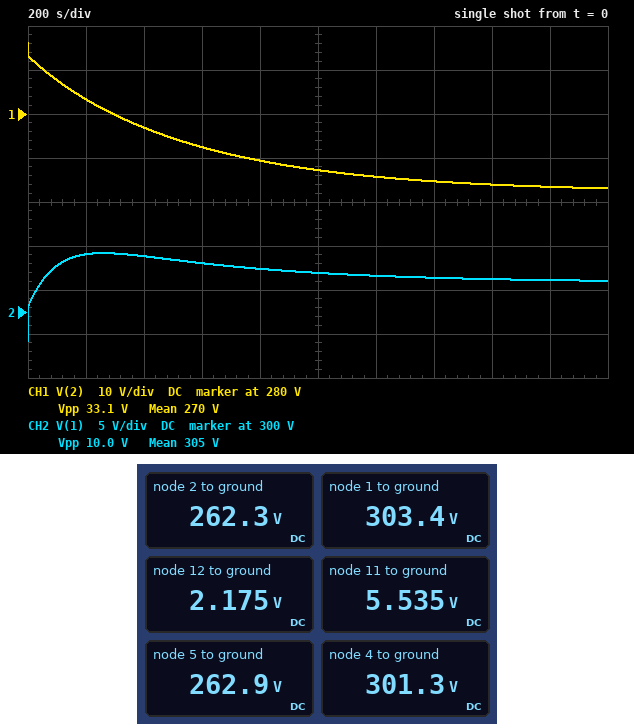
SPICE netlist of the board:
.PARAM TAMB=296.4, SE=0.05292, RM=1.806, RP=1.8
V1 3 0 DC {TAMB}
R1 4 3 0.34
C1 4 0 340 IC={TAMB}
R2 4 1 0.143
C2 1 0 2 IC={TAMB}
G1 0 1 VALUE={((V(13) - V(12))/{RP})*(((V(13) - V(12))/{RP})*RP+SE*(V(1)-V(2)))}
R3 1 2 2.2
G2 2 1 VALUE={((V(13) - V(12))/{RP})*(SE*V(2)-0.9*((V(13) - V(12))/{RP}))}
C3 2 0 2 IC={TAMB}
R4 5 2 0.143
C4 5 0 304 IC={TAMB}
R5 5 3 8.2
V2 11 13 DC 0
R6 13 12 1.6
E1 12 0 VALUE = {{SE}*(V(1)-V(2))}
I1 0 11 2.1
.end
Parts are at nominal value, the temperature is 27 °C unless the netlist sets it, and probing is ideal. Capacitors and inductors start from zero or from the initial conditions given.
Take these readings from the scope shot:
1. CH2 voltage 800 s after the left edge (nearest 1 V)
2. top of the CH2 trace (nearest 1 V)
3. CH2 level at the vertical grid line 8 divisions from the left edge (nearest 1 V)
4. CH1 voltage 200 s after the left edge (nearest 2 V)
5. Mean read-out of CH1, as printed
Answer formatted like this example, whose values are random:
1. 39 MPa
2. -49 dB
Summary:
1. 305 V
2. 307 V
3. 304 V
4. 284 V
5. 270 V
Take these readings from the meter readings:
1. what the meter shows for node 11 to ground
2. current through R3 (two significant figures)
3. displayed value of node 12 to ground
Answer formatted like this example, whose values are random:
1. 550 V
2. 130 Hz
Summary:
1. 5.535 V
2. 19 A
3. 2.175 V
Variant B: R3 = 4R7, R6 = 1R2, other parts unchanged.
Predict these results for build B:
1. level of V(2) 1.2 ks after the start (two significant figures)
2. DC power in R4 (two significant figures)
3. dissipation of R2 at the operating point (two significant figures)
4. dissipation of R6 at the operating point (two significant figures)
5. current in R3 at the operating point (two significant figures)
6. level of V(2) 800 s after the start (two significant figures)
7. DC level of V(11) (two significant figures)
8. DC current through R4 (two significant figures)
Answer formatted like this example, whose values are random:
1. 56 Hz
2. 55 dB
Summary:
1. 260 V
2. 4.4 W
3. 24 W
4. 5.3 W
5. 11 A
6. 270 V
7. 5.3 V
8. 5.6 A
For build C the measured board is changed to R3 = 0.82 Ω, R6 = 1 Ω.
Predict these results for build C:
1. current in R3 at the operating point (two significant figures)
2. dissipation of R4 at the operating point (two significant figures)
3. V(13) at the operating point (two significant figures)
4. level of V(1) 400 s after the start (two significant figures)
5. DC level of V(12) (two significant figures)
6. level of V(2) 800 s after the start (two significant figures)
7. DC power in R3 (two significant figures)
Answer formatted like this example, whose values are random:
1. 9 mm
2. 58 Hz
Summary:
1. 15 A
2. 220 mW
3. 2.8 V
4. 300 V
5. 660 mV
6. 290 V
7. 190 W
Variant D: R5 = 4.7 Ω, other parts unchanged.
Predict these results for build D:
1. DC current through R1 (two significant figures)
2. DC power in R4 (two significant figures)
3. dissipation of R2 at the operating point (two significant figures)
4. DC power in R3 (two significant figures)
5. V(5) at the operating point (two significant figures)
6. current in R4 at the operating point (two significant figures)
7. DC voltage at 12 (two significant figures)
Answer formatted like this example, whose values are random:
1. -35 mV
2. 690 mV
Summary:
1. 16 A
2. 5.4 W
3. 37 W
4. 640 W
5. 270 V
6. 6.1 A
7. 2.0 V
